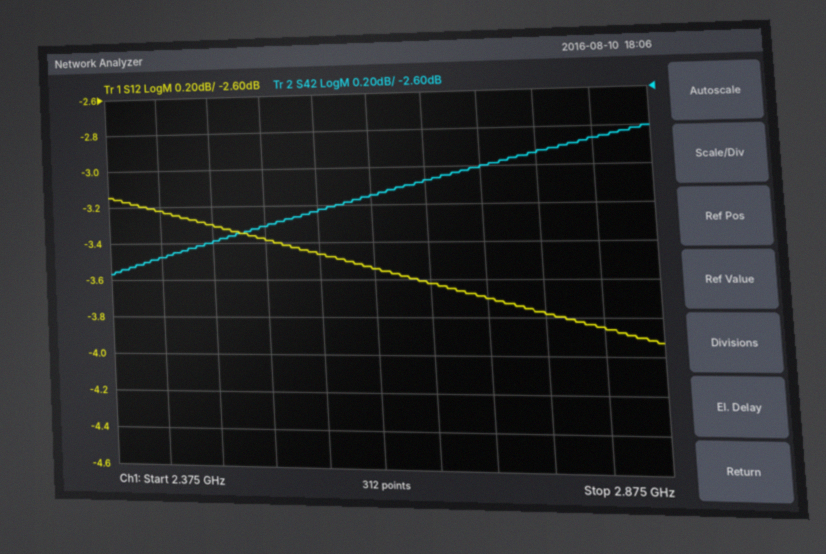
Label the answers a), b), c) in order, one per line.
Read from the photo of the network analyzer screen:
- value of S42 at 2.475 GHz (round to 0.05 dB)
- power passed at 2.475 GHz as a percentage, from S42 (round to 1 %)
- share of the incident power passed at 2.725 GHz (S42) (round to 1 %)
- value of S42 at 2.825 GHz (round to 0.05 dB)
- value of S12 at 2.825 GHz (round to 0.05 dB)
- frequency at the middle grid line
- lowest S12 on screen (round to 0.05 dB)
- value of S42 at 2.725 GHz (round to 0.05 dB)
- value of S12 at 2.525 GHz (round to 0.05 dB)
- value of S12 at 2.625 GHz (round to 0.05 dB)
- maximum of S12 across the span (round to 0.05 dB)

a) -3.40 dB
b) 46 %
c) 50 %
d) -2.85 dB
e) -3.85 dB
f) 2.625 GHz
g) -3.95 dB
h) -3.00 dB
i) -3.40 dB
j) -3.55 dB
k) -3.15 dB
